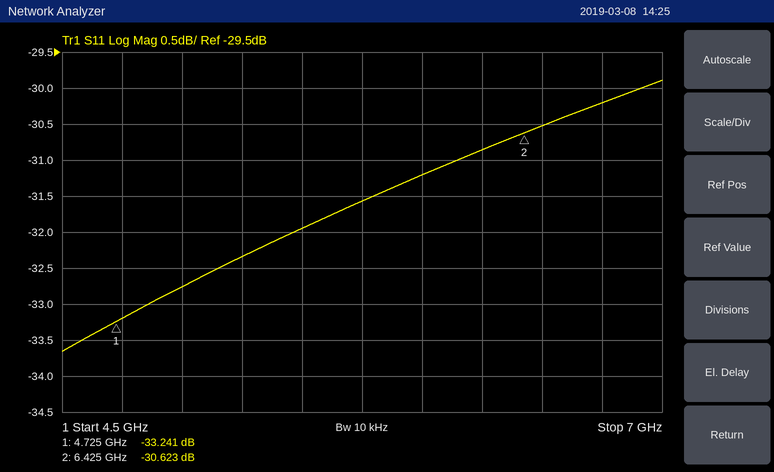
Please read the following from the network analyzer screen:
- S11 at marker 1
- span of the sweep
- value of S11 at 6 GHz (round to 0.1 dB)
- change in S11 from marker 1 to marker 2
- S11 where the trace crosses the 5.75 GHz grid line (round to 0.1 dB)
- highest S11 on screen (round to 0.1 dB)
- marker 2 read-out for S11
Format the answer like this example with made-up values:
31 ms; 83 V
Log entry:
-33.241 dB; 2.5 GHz; -31.2 dB; 2.618 dB; -31.6 dB; -29.9 dB; -30.623 dB
